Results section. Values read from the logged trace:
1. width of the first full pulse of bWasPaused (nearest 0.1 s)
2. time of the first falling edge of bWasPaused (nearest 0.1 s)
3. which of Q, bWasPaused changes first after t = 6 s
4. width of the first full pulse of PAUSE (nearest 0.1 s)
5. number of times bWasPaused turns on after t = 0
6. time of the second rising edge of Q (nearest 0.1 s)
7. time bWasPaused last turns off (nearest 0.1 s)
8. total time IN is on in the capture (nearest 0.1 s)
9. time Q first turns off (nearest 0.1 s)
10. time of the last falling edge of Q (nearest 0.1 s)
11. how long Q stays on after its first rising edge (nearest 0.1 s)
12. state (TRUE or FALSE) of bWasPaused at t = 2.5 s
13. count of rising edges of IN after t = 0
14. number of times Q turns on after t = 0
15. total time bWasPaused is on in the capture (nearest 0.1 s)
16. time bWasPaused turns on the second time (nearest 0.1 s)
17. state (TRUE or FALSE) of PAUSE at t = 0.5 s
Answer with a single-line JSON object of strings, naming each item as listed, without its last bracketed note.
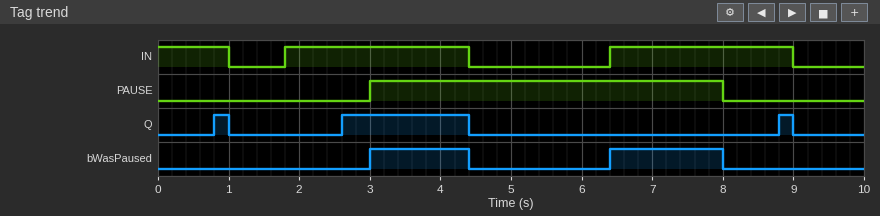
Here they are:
{"width of the first full pulse of bWasPaused": "1.4 s", "time of the first falling edge of bWasPaused": "4.4 s", "which of Q, bWasPaused changes first after t = 6 s": "bWasPaused", "width of the first full pulse of PAUSE": "5.0 s", "number of times bWasPaused turns on after t = 0": "2", "time of the second rising edge of Q": "2.6 s", "time bWasPaused last turns off": "8.0 s", "total time IN is on in the capture": "6.2 s", "time Q first turns off": "1.0 s", "time of the last falling edge of Q": "9.0 s", "how long Q stays on after its first rising edge": "0.2 s", "state (TRUE or FALSE) of bWasPaused at t = 2.5 s": "FALSE", "count of rising edges of IN after t = 0": "2", "number of times Q turns on after t = 0": "3", "total time bWasPaused is on in the capture": "3.0 s", "time bWasPaused turns on the second time": "6.4 s", "state (TRUE or FALSE) of PAUSE at t = 0.5 s": "FALSE"}
